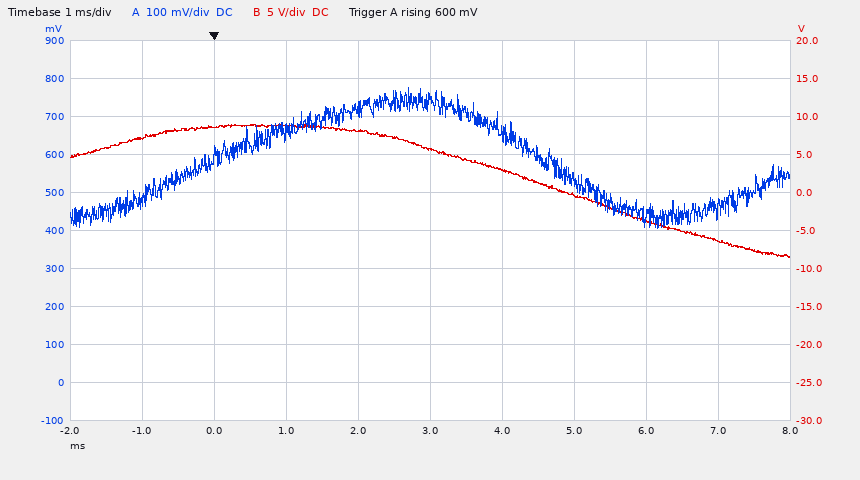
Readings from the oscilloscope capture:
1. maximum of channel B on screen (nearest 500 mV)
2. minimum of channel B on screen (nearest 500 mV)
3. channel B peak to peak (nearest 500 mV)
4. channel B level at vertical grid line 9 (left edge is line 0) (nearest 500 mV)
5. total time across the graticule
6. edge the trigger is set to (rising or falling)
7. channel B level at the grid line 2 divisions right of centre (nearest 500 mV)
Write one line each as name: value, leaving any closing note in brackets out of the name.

maximum of channel B on screen: 9.0 V
minimum of channel B on screen: -8.5 V
channel B peak to peak: 17.5 V
channel B level at vertical grid line 9 (left edge is line 0): -6.5 V
total time across the graticule: 10 ms
edge the trigger is set to: rising
channel B level at the grid line 2 divisions right of centre: -500 mV
